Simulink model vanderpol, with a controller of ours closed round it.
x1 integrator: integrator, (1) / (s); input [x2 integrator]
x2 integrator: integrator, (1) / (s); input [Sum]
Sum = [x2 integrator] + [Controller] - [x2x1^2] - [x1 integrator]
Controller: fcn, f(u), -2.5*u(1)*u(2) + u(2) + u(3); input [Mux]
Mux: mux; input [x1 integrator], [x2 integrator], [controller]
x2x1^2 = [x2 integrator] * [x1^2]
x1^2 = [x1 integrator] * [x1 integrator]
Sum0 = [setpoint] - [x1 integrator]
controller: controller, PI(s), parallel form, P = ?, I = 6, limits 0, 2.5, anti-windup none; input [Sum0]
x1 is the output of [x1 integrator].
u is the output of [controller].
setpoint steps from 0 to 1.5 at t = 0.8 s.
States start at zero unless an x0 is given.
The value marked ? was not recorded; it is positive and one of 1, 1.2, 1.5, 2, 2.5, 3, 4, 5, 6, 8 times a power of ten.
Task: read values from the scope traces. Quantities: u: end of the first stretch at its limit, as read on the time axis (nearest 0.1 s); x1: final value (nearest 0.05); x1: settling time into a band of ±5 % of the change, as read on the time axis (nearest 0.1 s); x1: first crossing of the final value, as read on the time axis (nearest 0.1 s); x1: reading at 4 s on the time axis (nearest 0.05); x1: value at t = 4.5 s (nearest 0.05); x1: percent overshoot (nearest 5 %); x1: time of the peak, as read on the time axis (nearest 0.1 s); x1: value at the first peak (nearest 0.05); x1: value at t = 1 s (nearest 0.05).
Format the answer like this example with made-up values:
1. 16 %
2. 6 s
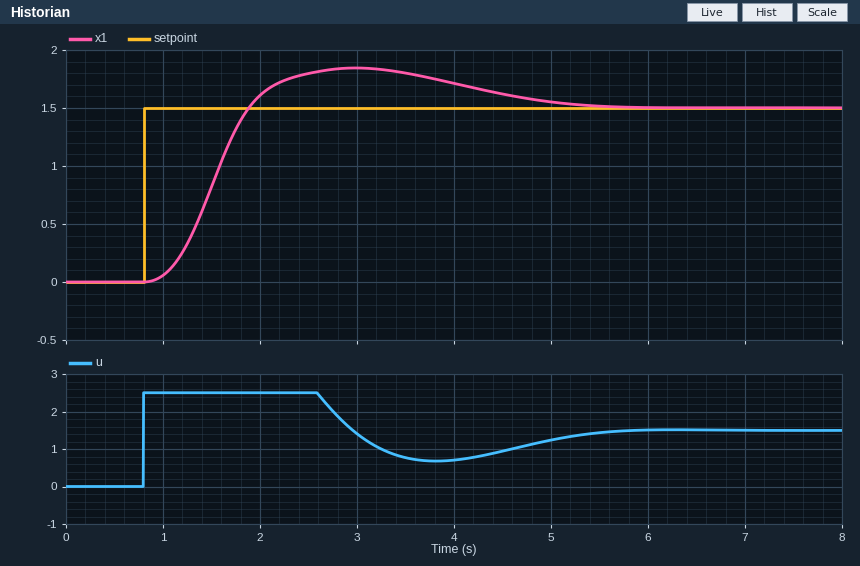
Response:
1. 2.6 s
2. 1.50
3. 4.8 s
4. 1.9 s
5. 1.70
6. 1.60
7. 25 %
8. 3.0 s
9. 1.85
10. 0.05
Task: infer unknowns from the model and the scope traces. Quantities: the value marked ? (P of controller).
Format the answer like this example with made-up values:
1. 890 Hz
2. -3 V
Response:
1. 8
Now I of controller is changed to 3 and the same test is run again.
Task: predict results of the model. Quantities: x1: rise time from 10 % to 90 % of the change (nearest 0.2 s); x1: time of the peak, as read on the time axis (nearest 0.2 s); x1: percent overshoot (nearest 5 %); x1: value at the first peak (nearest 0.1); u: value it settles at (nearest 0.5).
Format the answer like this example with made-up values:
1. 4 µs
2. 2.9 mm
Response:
1. 0.6 s
2. 2.4 s
3. 15 %
4. 1.7
5. 1.5
